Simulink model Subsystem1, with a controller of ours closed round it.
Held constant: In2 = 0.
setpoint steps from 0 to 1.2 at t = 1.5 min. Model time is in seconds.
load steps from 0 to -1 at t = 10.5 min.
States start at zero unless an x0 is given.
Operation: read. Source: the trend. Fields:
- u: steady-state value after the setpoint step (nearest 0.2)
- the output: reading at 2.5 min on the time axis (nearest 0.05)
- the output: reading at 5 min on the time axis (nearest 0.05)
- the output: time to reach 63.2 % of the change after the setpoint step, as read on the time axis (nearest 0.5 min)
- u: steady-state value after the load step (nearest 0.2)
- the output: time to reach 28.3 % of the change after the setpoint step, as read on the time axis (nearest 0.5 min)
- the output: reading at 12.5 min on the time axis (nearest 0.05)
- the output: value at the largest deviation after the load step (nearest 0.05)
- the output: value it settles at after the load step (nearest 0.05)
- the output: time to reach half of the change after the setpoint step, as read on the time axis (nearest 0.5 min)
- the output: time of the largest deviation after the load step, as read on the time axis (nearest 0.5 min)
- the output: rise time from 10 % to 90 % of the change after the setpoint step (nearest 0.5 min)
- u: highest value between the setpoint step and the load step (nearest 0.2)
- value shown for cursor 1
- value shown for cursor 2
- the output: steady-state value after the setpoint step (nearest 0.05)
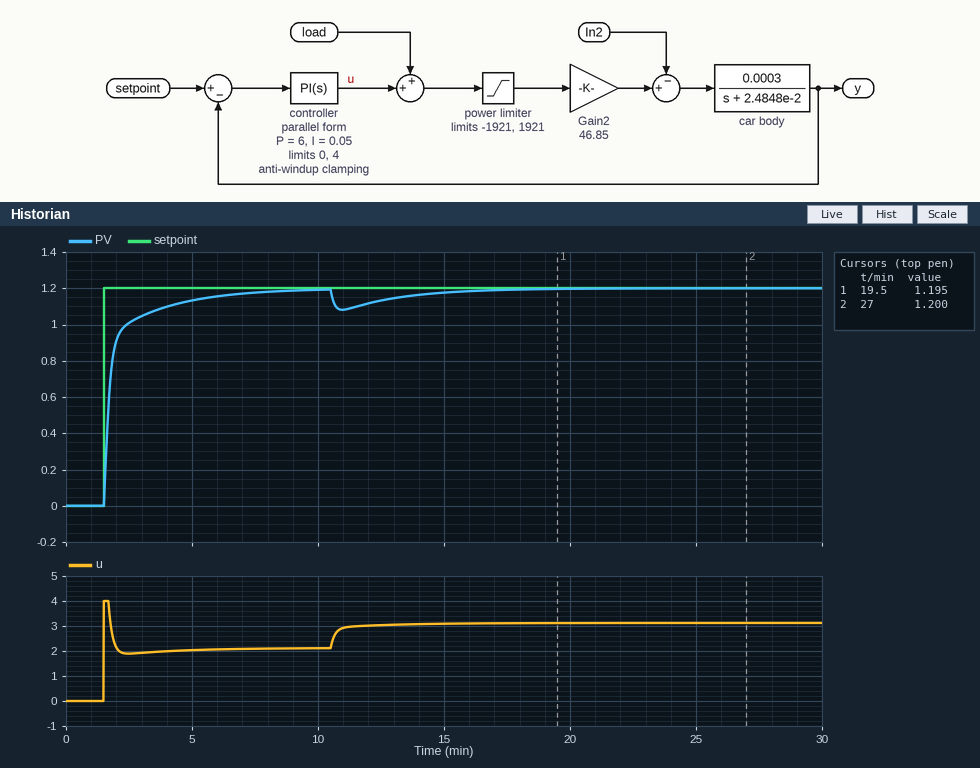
2.2
1.00
1.15
2.0 min
3.2
1.5 min
1.15
1.10
1.20
1.5 min
11.0 min
2.0 min
4.0
1.195
1.200
1.20
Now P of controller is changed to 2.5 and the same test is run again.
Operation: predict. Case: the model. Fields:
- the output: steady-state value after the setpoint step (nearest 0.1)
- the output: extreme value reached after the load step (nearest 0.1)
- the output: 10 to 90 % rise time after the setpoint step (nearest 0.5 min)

1.2
1.0
1.5 min
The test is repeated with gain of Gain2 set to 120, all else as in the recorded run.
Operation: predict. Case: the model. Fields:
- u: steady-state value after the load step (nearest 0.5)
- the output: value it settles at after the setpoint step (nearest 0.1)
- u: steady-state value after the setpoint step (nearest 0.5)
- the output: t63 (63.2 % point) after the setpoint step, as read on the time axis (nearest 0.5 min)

2.0
1.2
1.0
1.5 min
